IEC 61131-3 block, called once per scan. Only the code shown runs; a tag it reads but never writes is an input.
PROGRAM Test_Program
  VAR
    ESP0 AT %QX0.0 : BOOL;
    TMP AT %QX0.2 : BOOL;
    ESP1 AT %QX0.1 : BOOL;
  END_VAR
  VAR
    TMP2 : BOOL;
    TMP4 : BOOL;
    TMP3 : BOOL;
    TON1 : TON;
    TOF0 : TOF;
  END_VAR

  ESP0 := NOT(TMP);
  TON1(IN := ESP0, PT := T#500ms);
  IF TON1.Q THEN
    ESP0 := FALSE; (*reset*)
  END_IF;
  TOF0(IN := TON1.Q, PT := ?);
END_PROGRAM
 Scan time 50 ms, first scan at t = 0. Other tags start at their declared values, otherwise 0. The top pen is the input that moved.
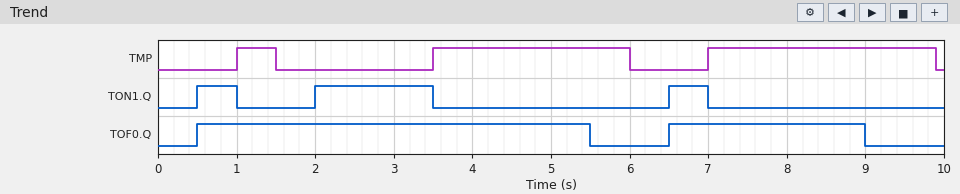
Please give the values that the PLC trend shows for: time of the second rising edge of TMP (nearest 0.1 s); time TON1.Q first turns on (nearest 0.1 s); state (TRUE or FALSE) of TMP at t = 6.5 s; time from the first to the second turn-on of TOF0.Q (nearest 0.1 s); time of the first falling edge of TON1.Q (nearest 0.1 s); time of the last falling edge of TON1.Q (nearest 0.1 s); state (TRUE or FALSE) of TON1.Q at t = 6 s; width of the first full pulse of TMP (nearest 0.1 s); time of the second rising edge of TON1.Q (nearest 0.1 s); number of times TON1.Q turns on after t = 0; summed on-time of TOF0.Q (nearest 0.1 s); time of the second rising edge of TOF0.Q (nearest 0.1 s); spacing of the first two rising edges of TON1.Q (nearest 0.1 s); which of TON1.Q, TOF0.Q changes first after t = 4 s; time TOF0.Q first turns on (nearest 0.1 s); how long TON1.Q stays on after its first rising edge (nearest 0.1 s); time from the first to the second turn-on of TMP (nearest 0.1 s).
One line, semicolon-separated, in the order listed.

3.5 s; 0.5 s; FALSE; 6.0 s; 1.0 s; 7.0 s; FALSE; 0.5 s; 2.0 s; 3; 7.5 s; 6.5 s; 1.5 s; TOF0.Q; 0.5 s; 0.5 s; 2.5 s
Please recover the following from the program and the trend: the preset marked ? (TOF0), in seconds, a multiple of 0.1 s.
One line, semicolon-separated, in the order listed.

2.0 s
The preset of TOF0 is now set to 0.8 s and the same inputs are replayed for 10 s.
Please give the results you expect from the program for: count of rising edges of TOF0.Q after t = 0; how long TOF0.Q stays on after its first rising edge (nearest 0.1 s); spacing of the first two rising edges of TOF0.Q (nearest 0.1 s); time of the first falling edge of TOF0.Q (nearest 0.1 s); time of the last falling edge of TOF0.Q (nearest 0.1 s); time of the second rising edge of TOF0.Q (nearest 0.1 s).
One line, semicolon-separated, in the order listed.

3; 1.3 s; 1.5 s; 1.8 s; 7.8 s; 2.0 s
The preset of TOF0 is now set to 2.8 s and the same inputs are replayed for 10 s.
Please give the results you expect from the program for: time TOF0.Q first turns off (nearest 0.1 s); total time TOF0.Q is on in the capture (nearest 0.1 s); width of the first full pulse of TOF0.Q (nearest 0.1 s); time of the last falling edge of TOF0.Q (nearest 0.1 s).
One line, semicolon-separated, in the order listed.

6.3 s; 9.1 s; 5.8 s; 9.8 s
